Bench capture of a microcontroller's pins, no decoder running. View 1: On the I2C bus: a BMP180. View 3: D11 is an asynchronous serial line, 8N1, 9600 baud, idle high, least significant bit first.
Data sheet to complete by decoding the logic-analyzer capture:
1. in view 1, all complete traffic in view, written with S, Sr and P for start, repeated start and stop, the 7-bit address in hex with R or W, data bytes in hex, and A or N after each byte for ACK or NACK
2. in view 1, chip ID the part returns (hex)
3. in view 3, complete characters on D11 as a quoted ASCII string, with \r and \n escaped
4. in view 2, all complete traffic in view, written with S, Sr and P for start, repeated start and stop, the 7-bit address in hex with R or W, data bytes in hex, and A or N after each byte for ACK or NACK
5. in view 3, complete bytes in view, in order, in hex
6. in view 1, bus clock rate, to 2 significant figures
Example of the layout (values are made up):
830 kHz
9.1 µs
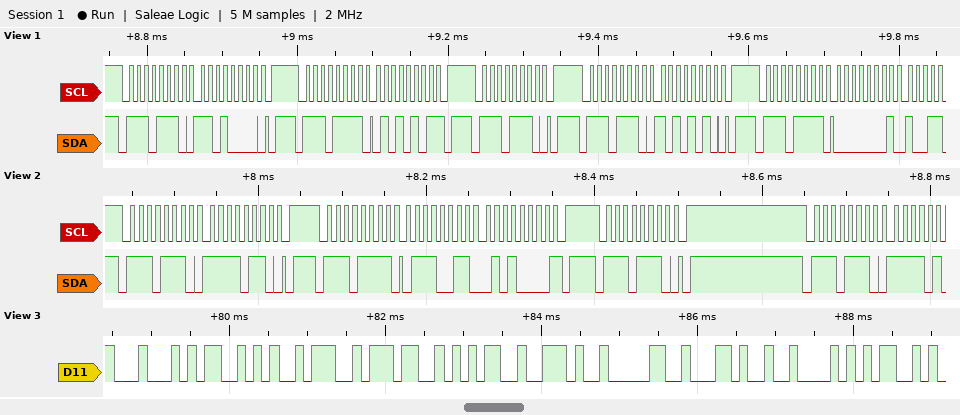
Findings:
S 77W A D0 A P S 77R A 55 N P S 77W A P S 77W A AA A P S 77R A 01 A
0x55
"DS:75.0,BM"
S 77W A F6 A P S 77R A 73 A 50 N P S 77W A P S 77W A
44 53 3A 37 35 2E 30 2C 42 4D
100 kHz
